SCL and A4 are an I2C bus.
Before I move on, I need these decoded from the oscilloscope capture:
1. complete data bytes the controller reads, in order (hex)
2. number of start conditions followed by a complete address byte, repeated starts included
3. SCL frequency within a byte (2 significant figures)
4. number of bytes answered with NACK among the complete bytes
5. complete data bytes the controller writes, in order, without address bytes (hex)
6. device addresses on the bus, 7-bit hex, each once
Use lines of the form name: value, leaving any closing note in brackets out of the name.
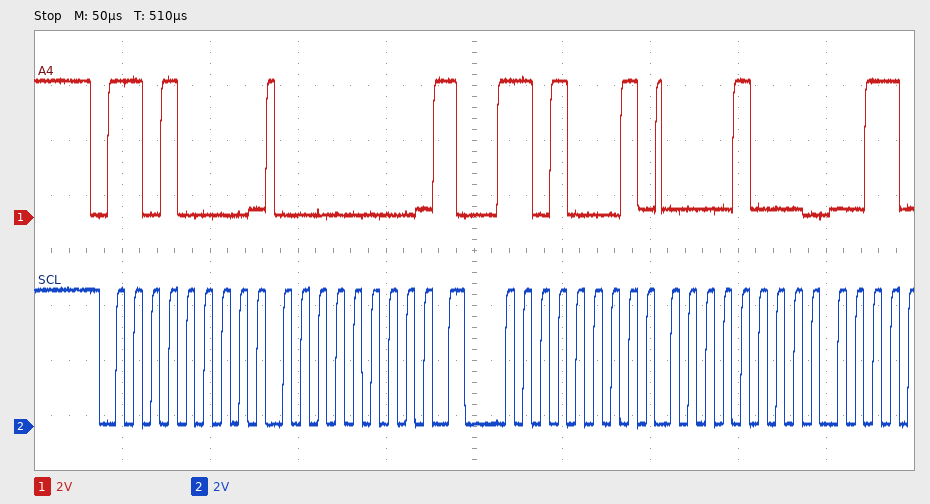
complete data bytes the controller reads, in order: 08
number of start conditions followed by a complete address byte, repeated starts included: 2
SCL frequency within a byte: 100 kHz
number of bytes answered with NACK among the complete bytes: 0
complete data bytes the controller writes, in order, without address bytes: 00
device addresses on the bus, 7-bit hex, each once: 0x68
